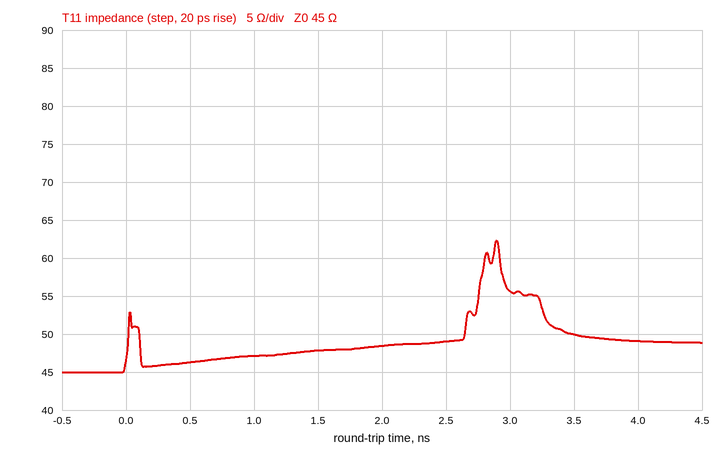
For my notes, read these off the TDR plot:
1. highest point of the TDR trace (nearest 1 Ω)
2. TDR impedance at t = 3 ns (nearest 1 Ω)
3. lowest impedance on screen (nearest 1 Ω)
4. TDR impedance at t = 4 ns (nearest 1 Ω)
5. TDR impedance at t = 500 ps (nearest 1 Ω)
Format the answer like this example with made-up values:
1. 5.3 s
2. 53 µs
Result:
1. 62 Ω
2. 56 Ω
3. 45 Ω
4. 49 Ω
5. 46 Ω
